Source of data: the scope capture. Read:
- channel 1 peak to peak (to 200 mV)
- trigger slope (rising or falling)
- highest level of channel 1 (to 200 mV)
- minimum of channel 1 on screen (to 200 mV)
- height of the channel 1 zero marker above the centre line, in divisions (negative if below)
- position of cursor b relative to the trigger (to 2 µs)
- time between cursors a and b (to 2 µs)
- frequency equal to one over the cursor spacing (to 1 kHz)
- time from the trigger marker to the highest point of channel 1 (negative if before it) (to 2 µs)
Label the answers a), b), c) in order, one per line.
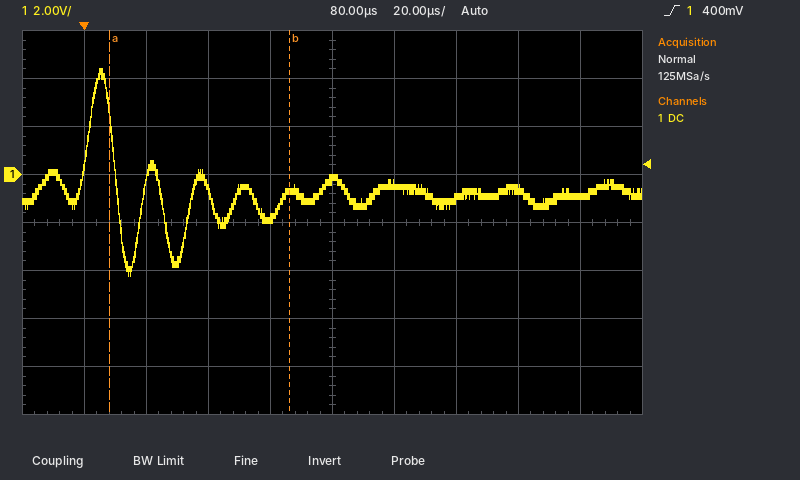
a) 8.6 V
b) rising
c) 4.4 V
d) -4.2 V
e) +1.0 div
f) +66 µs
g) 58 µs
h) 17 kHz
i) +6 µs
